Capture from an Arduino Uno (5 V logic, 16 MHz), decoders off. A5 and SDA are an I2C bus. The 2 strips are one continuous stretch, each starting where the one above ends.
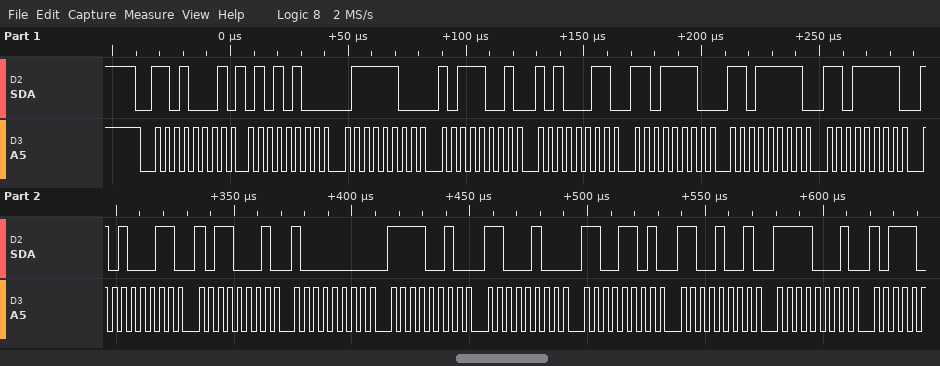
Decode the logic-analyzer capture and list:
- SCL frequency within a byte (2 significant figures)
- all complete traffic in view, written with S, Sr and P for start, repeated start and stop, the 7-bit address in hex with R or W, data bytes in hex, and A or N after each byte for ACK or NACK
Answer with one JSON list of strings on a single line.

["250 kHz", "S 68R A 54 A 7C A B9 A A3 A DE A DF A DF A A3 A B1 A 80 A F2 A C4 A CD A C9 A F1 A"]
